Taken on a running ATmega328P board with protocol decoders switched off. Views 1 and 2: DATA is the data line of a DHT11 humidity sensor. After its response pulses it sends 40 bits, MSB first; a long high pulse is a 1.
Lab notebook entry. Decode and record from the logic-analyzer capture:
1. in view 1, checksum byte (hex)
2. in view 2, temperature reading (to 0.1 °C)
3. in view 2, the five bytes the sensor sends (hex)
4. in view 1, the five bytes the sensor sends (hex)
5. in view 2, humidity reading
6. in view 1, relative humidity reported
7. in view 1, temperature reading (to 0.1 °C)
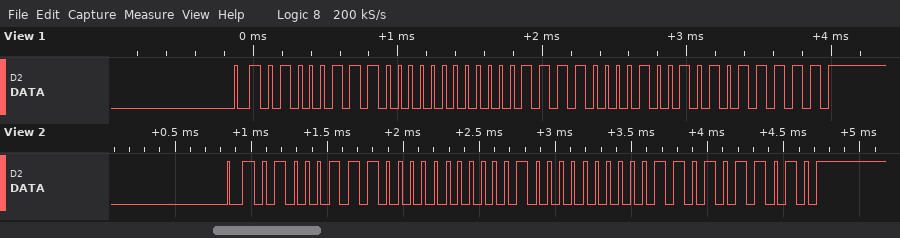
0x5F
16.3 °C
47 00 10 03 5A
47 00 0F 09 5F
71 %
71 %
15.9 °C
